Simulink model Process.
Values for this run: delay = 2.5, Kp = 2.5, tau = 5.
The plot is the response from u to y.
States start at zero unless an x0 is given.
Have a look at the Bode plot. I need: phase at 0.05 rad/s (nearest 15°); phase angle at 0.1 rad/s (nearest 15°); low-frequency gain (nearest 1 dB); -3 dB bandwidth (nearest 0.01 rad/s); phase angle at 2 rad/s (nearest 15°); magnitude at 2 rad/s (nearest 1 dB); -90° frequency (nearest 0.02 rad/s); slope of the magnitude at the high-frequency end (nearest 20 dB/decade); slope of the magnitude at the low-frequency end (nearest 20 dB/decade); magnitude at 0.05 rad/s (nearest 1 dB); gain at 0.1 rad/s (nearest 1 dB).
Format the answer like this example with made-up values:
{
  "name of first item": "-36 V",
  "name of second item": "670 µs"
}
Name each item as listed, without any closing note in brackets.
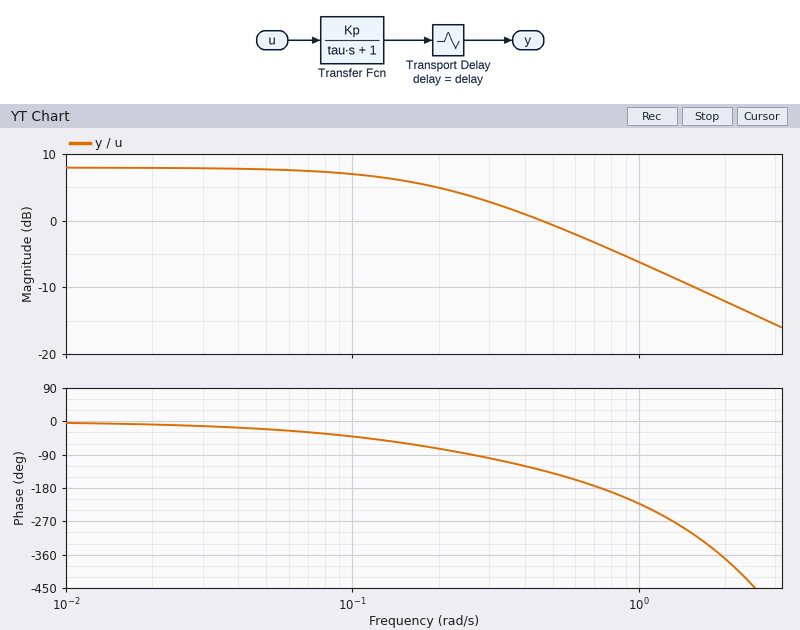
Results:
{
  "phase at 0.05 rad/s": "-15°",
  "phase angle at 0.1 rad/s": "-45°",
  "low-frequency gain": "8 dB",
  "-3 dB bandwidth": "0.20 rad/s",
  "phase angle at 2 rad/s": "-375°",
  "magnitude at 2 rad/s": "-12 dB",
  "-90° frequency": "0.26 rad/s",
  "slope of the magnitude at the high-frequency end": "-20 dB/decade",
  "slope of the magnitude at the low-frequency end": "0 dB/decade",
  "magnitude at 0.05 rad/s": "8 dB",
  "gain at 0.1 rad/s": "7 dB"
}
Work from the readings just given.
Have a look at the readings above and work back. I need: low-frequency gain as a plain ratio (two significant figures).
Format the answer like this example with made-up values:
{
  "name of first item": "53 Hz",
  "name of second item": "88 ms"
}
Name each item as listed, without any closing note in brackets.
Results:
{
  "low-frequency gain as a plain ratio": "2.5"
}
